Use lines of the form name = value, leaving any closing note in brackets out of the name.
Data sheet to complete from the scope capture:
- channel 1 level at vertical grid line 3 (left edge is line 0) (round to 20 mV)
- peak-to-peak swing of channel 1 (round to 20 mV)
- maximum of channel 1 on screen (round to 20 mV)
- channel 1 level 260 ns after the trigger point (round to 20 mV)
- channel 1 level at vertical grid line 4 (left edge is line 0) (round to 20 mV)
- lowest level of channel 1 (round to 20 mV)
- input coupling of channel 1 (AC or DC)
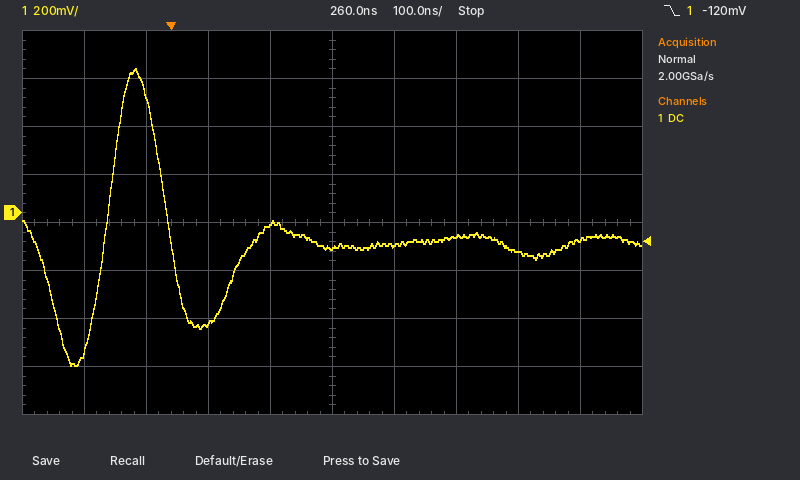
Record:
channel 1 level at vertical grid line 3 (left edge is line 0) = -460 mV
peak-to-peak swing of channel 1 = 1.24 V
maximum of channel 1 on screen = 600 mV
channel 1 level 260 ns after the trigger point = -140 mV
channel 1 level at vertical grid line 4 (left edge is line 0) = -40 mV
lowest level of channel 1 = -640 mV
input coupling of channel 1 = DC
